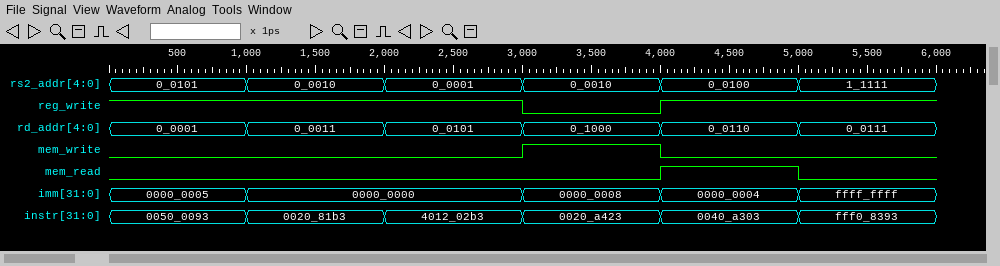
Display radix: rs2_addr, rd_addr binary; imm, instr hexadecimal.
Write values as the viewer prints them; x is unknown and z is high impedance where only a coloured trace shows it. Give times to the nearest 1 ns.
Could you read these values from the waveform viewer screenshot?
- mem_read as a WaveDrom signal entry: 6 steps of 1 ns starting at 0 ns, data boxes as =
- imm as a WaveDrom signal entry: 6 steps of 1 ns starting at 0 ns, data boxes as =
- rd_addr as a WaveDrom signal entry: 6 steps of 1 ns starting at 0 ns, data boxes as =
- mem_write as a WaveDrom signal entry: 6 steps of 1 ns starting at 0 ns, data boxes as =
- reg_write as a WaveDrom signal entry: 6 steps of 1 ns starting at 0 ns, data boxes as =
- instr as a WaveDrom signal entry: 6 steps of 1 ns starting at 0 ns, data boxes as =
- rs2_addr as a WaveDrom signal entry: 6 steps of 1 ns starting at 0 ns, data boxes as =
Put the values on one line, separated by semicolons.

{name: 'mem_read', wave: '0...10'}; {name: 'imm', wave: '==.===', data: '0000_0005 0000_0000 0000_0008 0000_0004 ffff_ffff'}; {name: 'rd_addr', wave: '======', data: '0_0001 0_0011 0_0101 0_1000 0_0110 0_0111'}; {name: 'mem_write', wave: '0..10.'}; {name: 'reg_write', wave: '1..01.'}; {name: 'instr', wave: '======', data: '0050_0093 0020_81b3 4012_02b3 0020_a423 0040_a303 fff0_8393'}; {name: 'rs2_addr', wave: '======', data: '0_0101 0_0010 0_0001 0_0010 0_0100 1_1111'}
